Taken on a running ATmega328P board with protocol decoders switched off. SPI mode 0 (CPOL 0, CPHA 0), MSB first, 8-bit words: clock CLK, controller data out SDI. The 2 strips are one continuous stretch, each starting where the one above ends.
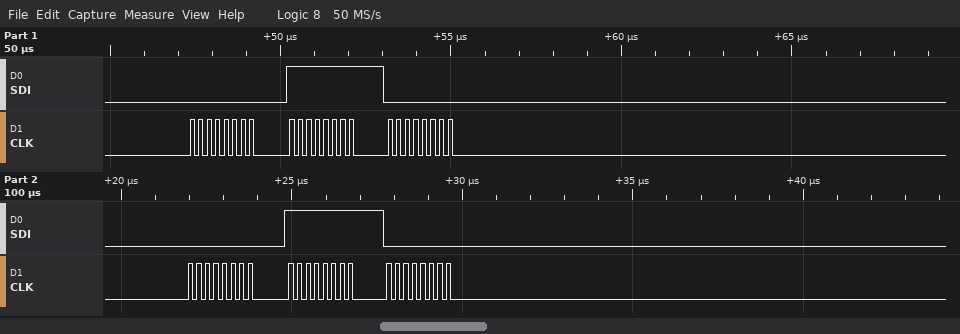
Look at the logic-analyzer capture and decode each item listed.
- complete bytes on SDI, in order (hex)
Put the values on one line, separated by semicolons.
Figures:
0x00 0xFF 0x00 0x00 0xFF 0x00
